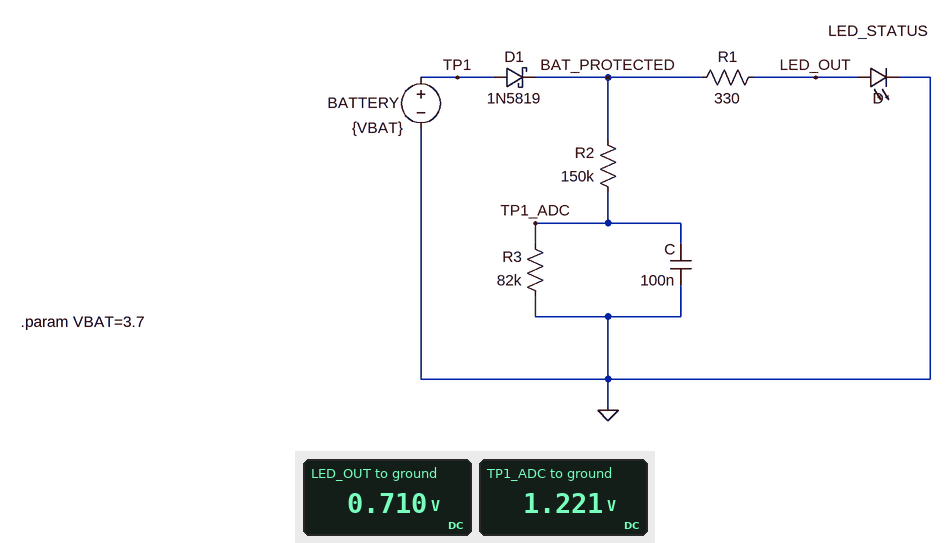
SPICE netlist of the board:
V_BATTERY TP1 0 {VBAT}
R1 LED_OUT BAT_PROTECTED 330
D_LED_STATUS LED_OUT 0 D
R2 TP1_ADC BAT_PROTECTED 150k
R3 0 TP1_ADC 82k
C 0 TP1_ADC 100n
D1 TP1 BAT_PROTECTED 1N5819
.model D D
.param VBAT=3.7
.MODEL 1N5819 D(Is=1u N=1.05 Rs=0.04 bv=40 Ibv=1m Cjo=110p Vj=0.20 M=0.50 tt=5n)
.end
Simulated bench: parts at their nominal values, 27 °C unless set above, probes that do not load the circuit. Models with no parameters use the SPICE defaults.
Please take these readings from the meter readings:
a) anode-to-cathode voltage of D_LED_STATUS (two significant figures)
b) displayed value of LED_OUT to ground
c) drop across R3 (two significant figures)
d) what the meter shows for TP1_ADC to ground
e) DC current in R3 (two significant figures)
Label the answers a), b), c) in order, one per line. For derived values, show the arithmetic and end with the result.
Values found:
a) 710 mV = 710 mV
b) 0.710 V
c) 1.221 V = 1.2 V
d) 1.221 V
e) (1.221 V) / 82 kΩ = 15 µA
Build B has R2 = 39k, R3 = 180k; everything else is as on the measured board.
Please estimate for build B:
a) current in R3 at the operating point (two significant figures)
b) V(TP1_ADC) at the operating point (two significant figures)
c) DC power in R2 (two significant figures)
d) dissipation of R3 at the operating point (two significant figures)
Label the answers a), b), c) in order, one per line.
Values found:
a) 16 µA
b) 2.8 V
c) 9.7 µW
d) 45 µW
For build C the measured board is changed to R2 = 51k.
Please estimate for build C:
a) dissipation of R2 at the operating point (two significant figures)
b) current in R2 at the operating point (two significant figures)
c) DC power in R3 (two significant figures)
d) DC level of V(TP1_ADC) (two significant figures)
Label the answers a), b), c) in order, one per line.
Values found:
a) 34 µW
b) 26 µA
c) 55 µW
d) 2.1 V
